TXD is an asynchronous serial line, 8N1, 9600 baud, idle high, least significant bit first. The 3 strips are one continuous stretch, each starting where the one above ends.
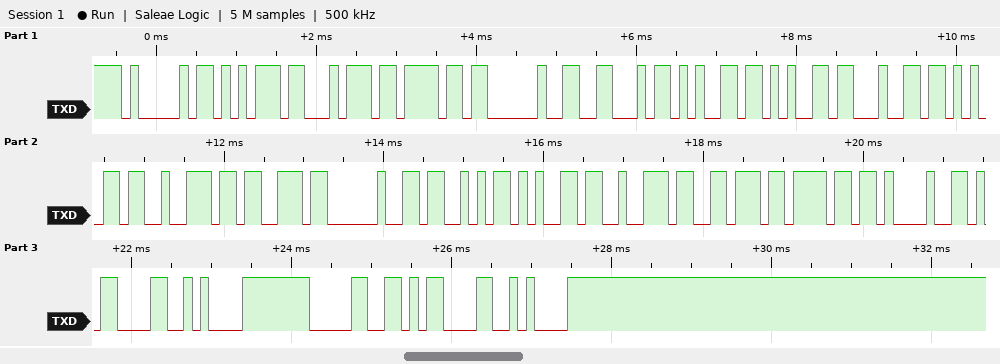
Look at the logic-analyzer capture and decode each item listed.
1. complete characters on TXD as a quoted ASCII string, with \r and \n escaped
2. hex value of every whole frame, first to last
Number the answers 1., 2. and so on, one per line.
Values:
1. "Auto Feeders Servo!\r\n0\r\n"
2. 41 75 74 6F 20 46 65 65 64 65 72 73 20 53 65 72 76 6F 21 0D 0A 30 0D 0A
